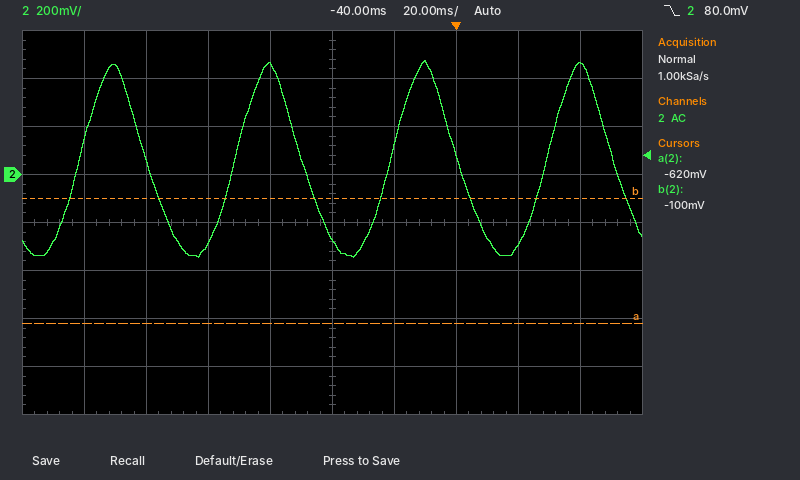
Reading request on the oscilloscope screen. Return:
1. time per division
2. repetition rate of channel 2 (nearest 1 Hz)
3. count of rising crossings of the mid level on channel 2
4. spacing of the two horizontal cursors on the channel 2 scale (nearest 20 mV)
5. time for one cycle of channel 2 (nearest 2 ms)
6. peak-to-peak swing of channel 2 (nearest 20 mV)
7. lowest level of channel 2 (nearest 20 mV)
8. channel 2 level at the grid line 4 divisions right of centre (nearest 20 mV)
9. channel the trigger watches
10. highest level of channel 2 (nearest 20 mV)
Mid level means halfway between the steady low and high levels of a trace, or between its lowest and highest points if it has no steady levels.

20 ms
20 Hz
4
520 mV
50 ms
820 mV
-340 mV
460 mV
channel 2
480 mV
